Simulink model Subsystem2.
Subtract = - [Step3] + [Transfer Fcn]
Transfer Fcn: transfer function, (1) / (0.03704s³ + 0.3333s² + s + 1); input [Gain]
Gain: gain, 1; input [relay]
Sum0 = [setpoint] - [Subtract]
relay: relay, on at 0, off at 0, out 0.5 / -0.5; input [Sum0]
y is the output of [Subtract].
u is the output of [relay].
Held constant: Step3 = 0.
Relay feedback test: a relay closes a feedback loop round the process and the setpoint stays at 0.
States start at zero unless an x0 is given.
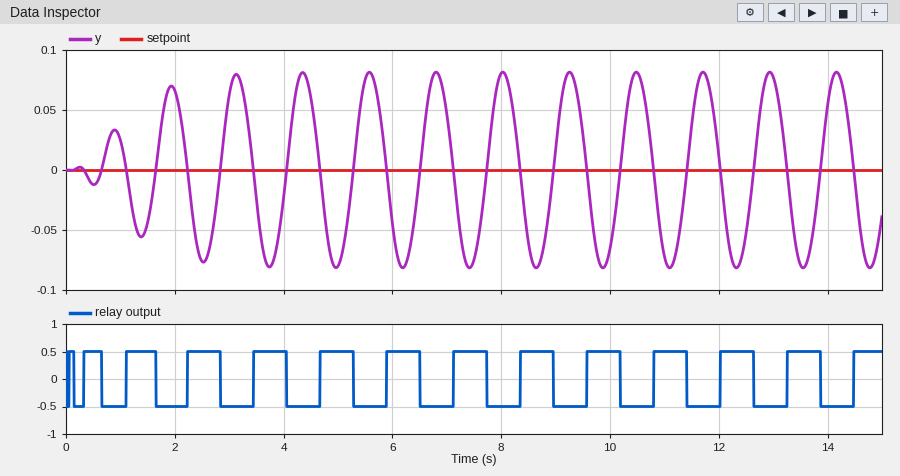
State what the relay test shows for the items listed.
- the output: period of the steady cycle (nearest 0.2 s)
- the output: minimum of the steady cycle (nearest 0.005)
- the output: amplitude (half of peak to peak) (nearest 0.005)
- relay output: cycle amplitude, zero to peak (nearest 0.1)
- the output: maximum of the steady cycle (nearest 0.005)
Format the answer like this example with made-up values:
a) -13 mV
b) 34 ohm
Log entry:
a) 1.2 s
b) -0.080
c) 0.080
d) 0.5
e) 0.080
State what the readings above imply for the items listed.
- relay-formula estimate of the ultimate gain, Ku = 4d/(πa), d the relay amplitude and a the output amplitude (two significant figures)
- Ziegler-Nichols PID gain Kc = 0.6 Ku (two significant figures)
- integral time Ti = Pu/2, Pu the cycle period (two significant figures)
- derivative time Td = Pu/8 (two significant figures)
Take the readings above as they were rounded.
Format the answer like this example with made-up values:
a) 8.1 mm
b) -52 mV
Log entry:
a) 8.0
b) 4.8
c) 0.60 s
d) 0.15 s
